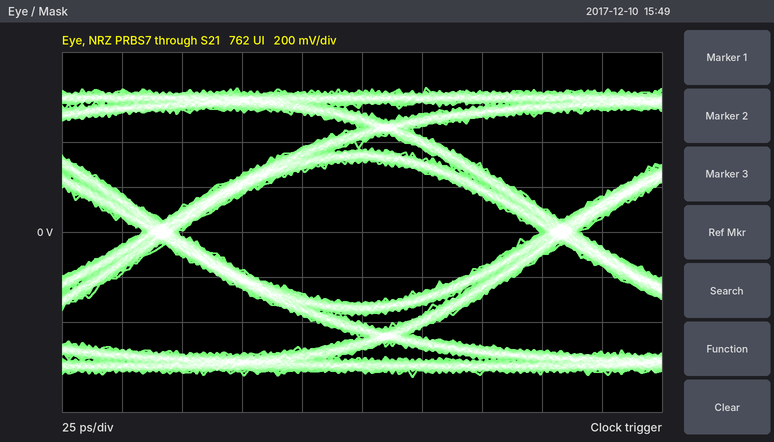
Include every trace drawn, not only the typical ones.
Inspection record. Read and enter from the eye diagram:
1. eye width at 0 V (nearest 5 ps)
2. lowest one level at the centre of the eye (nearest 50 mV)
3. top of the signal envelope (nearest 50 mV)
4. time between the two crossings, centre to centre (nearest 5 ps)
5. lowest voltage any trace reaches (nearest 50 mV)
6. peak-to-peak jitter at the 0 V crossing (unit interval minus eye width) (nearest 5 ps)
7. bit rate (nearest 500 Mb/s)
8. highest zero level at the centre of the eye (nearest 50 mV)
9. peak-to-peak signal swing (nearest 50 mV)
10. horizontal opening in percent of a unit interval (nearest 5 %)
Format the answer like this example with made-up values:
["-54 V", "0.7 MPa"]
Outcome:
["150 ps", "300 mV", "650 mV", "165 ps", "-650 mV", "15 ps", "6.0 Gb/s", "-300 mV", "1.30 V", "90 %"]
